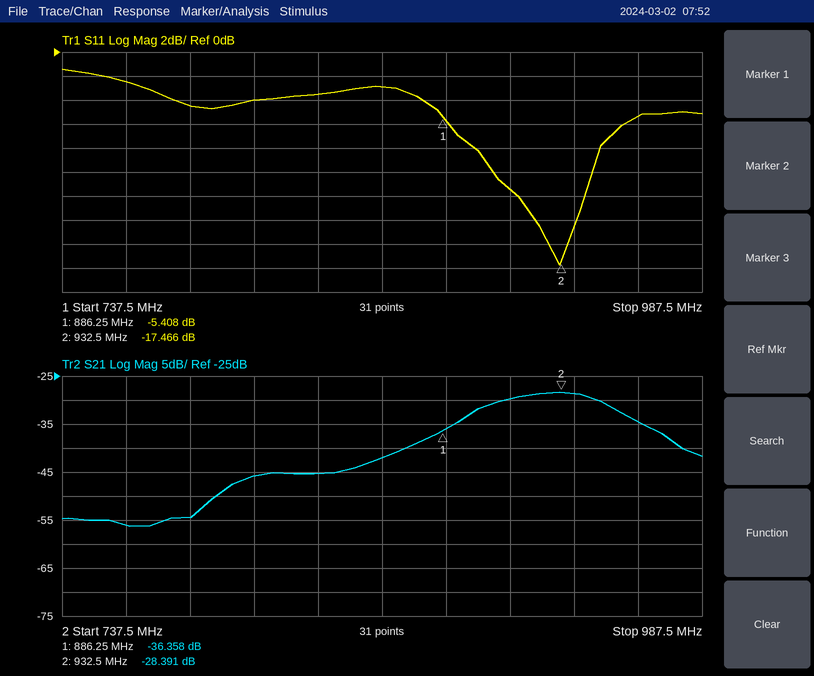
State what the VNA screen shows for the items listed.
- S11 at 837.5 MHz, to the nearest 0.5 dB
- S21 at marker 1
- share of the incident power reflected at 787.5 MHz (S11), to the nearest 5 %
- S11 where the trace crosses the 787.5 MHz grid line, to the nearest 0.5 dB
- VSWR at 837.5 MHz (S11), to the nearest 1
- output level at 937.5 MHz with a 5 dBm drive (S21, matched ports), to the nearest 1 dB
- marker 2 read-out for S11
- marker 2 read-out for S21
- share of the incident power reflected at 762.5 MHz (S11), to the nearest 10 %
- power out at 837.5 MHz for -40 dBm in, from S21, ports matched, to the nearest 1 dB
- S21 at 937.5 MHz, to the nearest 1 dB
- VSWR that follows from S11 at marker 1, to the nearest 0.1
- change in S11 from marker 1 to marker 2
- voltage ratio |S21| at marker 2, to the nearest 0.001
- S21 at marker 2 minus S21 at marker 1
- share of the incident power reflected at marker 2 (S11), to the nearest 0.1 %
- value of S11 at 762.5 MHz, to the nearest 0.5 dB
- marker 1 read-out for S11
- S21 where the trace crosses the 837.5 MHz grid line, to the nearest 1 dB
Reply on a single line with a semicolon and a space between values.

-3.5 dB; -36.358 dB; 35 %; -4.5 dB; 5; -24 dBm; -17.466 dB; -28.391 dB; 60 %; -85 dBm; -29 dB; 3.3; -12.058 dB; 0.038; 7.967 dB; 1.8 %; -2.5 dB; -5.408 dB; -45 dB
